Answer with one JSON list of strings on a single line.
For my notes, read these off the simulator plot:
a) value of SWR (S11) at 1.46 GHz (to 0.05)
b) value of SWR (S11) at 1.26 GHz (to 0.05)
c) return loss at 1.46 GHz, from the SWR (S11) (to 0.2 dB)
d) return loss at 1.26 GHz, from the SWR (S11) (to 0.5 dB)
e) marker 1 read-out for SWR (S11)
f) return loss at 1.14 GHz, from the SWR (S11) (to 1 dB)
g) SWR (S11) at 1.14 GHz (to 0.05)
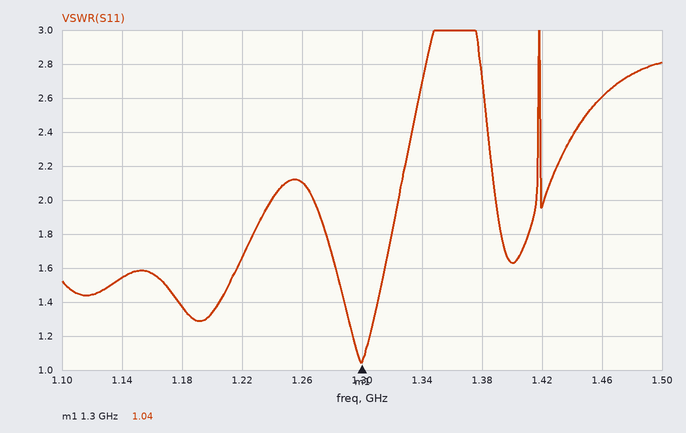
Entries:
["2.60", "2.10", "7.0 dB", "9.0 dB", "1.04", "13 dB", "1.55"]
